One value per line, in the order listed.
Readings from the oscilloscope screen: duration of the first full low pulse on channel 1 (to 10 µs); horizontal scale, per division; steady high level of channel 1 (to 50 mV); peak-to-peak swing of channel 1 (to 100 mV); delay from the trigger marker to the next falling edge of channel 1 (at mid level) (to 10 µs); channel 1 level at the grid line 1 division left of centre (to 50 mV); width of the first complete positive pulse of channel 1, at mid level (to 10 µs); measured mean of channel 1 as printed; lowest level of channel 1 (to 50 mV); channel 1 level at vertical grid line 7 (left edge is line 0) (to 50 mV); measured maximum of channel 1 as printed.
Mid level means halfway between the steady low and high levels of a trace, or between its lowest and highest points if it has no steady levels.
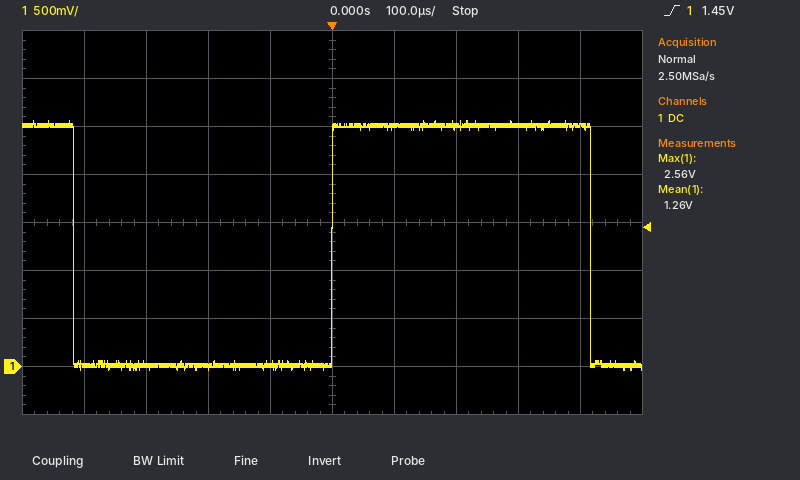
420 µs
100 µs
2.50 V
2.60 V
420 µs
50 mV
420 µs
1.26 V
-50 mV
2.50 V
2.56 V
